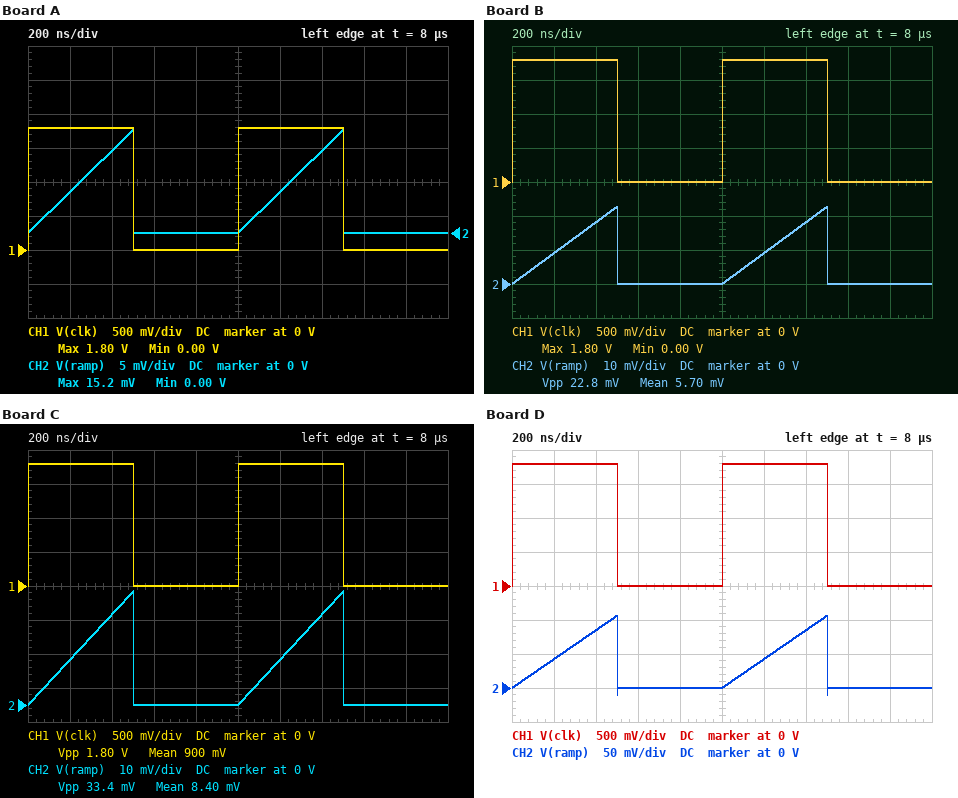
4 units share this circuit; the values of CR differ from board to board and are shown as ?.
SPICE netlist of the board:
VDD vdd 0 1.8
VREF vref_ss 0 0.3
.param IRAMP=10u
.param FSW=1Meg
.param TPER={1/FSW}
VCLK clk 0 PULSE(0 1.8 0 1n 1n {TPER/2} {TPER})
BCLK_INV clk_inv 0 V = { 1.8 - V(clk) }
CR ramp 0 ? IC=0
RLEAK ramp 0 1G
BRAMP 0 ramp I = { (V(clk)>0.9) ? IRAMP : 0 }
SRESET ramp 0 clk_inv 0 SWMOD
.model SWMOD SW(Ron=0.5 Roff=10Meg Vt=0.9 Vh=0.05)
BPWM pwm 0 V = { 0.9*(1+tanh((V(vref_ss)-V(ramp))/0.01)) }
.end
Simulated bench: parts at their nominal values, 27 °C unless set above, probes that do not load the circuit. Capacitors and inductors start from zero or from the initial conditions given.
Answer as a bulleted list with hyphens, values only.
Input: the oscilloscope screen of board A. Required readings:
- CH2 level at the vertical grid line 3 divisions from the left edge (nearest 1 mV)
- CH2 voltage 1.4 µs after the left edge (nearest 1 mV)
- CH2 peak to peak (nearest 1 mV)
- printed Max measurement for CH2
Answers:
- 0 V
- 12 mV
- 15 mV
- 15.2 mV
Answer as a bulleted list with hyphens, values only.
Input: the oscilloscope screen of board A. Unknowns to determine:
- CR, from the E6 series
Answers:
- 330 pF
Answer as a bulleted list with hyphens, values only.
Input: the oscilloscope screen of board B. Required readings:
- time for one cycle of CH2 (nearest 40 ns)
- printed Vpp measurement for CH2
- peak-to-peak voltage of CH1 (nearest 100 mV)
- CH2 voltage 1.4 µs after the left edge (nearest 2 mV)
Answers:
- 1.00 µs
- 22.8 mV
- 1.8 V
- 18 mV
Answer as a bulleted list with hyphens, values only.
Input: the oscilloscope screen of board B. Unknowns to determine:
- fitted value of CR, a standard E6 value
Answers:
- 220 pF
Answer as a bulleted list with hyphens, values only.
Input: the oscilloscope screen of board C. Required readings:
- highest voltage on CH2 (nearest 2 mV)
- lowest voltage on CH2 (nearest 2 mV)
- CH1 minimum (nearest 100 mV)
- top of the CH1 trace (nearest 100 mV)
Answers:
- 34 mV
- 0 V
- 0 V
- 1.8 V
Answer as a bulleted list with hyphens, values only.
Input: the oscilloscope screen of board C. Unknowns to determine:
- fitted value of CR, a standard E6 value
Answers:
- 150 pF
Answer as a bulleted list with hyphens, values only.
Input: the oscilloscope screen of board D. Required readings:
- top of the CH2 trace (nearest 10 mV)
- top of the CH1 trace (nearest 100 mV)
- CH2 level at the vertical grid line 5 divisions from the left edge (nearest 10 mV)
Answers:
- 110 mV
- 1.8 V
- 0 V
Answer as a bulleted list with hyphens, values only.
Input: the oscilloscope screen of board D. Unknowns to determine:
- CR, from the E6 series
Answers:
- 47 pF
